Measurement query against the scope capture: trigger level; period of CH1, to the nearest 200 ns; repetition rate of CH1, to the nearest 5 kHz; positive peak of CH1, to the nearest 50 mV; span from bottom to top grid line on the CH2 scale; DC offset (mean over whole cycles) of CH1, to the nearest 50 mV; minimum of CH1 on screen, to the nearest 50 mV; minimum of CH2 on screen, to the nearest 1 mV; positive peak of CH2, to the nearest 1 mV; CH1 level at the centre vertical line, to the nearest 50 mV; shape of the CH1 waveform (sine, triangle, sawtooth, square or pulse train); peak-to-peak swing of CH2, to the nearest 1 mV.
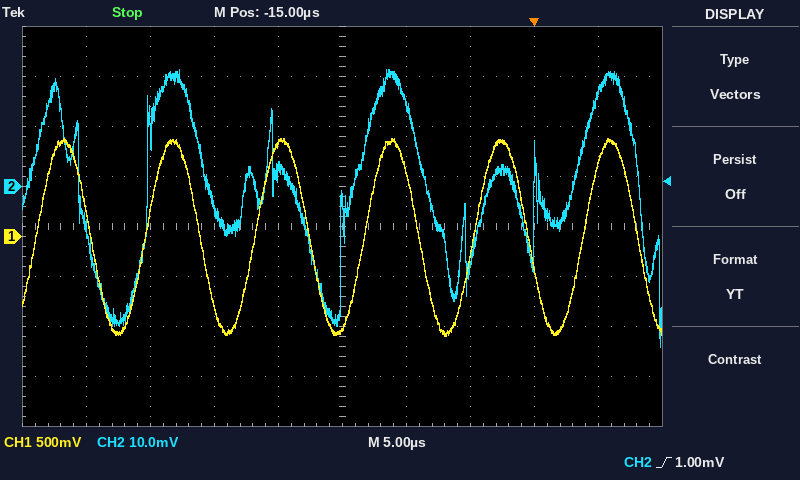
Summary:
1.00 mV
8.6 µs
115 kHz
1.00 V
80 mV
0 mV
-1.00 V
-32 mV
23 mV
-900 mV
sine
55 mV
